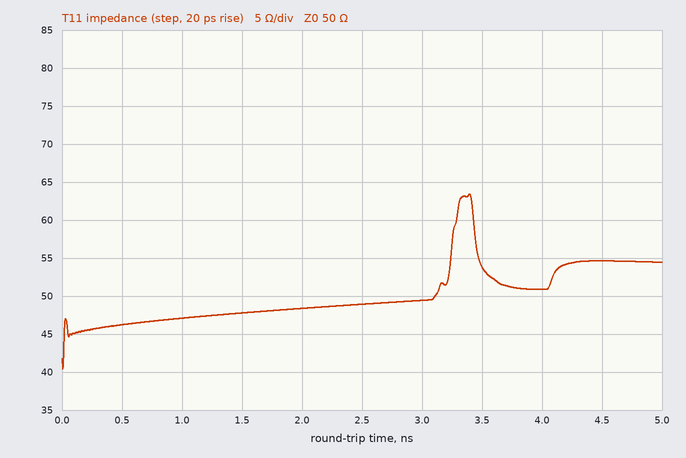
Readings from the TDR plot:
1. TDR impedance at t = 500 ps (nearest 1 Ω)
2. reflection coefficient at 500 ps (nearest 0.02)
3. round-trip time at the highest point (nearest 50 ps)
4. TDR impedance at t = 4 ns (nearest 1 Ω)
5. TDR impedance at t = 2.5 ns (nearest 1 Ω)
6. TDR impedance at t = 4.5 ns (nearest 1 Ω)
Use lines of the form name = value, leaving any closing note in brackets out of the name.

TDR impedance at t = 500 ps = 46 Ω
reflection coefficient at 500 ps = -0.04
round-trip time at the highest point = 3.40 ns
TDR impedance at t = 4 ns = 51 Ω
TDR impedance at t = 2.5 ns = 49 Ω
TDR impedance at t = 4.5 ns = 55 Ω
